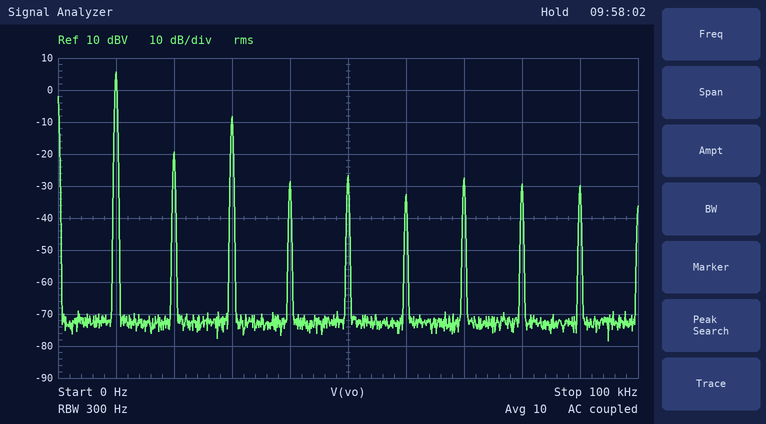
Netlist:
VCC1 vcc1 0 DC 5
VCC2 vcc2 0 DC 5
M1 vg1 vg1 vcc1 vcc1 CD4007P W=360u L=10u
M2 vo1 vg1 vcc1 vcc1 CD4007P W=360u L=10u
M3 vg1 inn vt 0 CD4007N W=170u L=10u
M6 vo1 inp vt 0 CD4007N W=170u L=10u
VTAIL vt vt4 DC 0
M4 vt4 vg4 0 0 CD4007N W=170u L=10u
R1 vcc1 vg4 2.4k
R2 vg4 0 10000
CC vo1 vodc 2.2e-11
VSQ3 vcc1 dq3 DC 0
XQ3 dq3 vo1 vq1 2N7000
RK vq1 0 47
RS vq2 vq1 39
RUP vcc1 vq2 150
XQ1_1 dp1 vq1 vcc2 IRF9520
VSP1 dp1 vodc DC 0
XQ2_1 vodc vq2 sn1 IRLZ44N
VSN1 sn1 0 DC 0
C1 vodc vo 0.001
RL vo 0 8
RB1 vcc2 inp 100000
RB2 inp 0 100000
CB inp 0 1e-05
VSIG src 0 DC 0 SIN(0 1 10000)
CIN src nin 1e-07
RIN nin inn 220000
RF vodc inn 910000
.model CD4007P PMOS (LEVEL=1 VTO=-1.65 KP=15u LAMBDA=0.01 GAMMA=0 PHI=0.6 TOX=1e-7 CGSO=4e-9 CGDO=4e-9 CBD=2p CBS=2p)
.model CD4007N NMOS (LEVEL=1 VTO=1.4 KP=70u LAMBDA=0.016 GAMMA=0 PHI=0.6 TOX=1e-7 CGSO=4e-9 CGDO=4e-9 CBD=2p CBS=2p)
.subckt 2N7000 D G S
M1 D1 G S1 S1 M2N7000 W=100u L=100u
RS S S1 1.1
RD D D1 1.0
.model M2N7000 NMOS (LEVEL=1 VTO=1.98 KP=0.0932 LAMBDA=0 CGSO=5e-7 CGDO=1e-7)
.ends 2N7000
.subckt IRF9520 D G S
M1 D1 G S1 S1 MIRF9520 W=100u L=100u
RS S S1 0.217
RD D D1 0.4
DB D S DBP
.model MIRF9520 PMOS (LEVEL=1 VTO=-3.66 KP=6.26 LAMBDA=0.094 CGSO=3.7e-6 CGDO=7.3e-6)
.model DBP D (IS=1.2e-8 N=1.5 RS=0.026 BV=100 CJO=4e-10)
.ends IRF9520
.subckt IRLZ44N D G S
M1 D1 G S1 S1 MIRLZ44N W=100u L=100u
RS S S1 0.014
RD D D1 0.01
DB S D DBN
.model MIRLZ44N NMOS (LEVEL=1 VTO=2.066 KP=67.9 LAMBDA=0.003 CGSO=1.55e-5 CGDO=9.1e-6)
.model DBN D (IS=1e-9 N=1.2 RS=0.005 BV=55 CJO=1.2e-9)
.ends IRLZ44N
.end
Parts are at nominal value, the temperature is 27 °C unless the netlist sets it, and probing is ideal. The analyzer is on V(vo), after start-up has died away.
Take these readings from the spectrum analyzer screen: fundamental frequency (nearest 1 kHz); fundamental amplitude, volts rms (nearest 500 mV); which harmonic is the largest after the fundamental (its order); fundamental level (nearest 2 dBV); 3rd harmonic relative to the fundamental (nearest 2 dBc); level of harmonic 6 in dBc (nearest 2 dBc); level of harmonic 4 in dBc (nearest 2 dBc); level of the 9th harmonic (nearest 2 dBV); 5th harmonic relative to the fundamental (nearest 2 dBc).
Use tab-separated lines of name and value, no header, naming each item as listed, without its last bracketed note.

fundamental frequency	10 kHz
fundamental amplitude, volts rms	2.0 V
which harmonic is the largest after the fundamental	3
fundamental level	6 dBV
3rd harmonic relative to the fundamental	-14 dBc
level of harmonic 6 in dBc	-38 dBc
level of harmonic 4 in dBc	-34 dBc
level of the 9th harmonic	-30 dBV
5th harmonic relative to the fundamental	-32 dBc
